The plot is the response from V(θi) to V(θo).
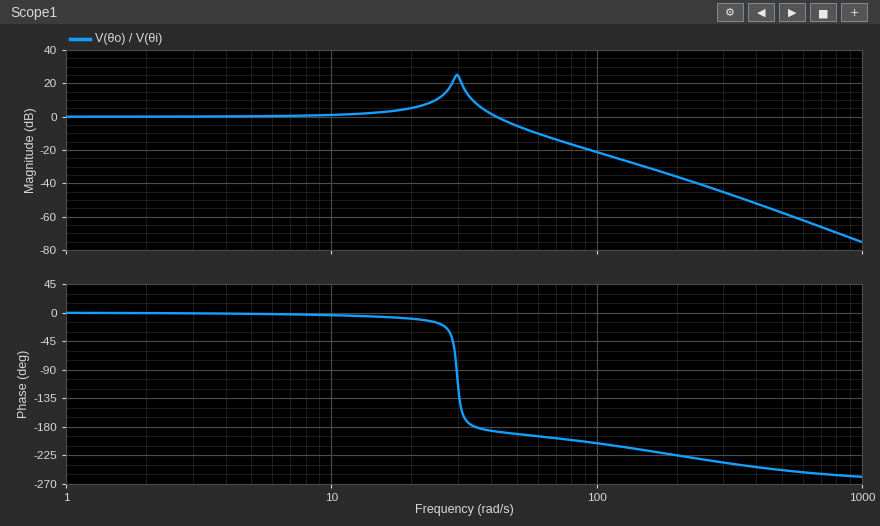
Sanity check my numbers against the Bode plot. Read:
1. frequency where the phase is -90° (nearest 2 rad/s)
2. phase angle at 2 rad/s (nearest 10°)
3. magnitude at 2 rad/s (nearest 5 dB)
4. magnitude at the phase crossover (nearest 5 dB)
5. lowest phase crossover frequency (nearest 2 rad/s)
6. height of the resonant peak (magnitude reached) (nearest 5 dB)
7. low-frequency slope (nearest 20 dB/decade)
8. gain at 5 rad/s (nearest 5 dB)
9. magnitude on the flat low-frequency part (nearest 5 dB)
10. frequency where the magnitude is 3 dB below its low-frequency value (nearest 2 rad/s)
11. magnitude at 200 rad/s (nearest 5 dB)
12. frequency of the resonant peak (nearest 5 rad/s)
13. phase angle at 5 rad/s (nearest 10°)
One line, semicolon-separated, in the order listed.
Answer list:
30 rad/s; 0°; 0 dB; 10 dB; 34 rad/s; 25 dB; 0 dB/decade; 0 dB; 0 dB; 46 rad/s; -35 dB; 30 rad/s; 0°
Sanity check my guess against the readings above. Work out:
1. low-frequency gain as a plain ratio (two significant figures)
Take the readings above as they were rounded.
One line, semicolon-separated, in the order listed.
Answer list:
1.0
